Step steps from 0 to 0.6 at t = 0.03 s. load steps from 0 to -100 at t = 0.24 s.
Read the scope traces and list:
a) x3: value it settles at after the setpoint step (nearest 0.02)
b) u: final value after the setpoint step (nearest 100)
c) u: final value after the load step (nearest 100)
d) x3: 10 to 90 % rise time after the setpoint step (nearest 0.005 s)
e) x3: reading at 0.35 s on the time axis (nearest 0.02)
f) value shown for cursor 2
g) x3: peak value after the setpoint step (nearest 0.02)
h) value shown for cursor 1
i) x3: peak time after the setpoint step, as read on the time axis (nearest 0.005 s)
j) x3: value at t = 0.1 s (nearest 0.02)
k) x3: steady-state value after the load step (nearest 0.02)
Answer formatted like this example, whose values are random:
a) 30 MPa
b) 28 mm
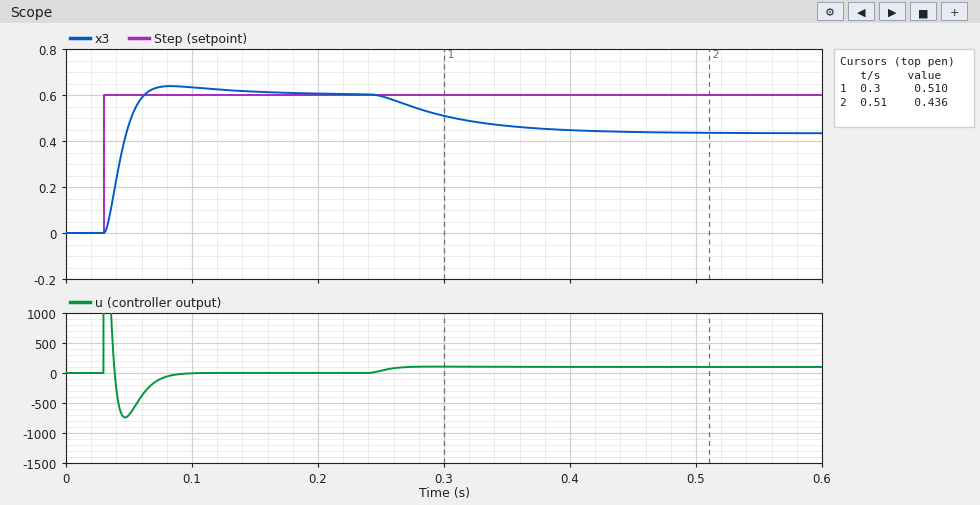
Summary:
a) 0.60
b) 0
c) 100
d) 0.020 s
e) 0.46
f) 0.436
g) 0.64
h) 0.510
i) 0.085 s
j) 0.64
k) 0.44
